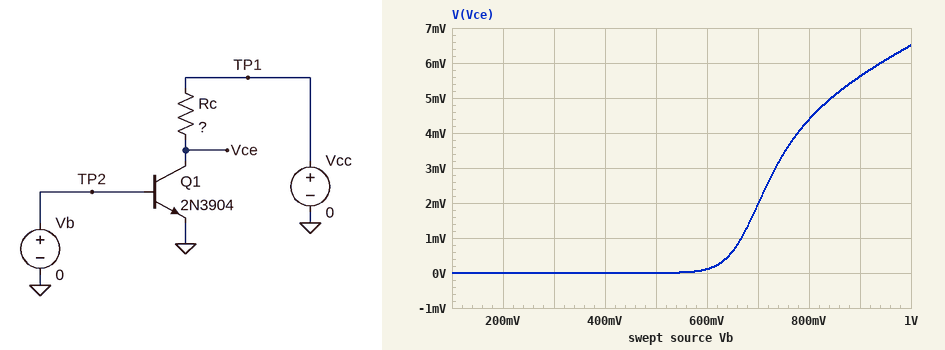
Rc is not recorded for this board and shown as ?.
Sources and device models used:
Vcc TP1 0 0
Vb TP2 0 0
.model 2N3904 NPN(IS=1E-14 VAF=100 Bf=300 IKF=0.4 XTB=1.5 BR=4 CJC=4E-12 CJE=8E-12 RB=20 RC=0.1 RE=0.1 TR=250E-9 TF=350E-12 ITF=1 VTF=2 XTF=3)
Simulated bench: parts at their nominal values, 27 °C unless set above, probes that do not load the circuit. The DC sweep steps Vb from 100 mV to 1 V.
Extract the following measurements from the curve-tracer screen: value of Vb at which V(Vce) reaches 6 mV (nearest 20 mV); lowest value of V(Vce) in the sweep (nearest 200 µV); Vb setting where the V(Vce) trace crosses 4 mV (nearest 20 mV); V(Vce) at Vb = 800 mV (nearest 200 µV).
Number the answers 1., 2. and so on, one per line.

1. 940 mV
2. 0 V
3. 780 mV
4. 4.4 mV
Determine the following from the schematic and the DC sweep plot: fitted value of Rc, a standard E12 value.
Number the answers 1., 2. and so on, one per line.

1. 3.9 Ω
